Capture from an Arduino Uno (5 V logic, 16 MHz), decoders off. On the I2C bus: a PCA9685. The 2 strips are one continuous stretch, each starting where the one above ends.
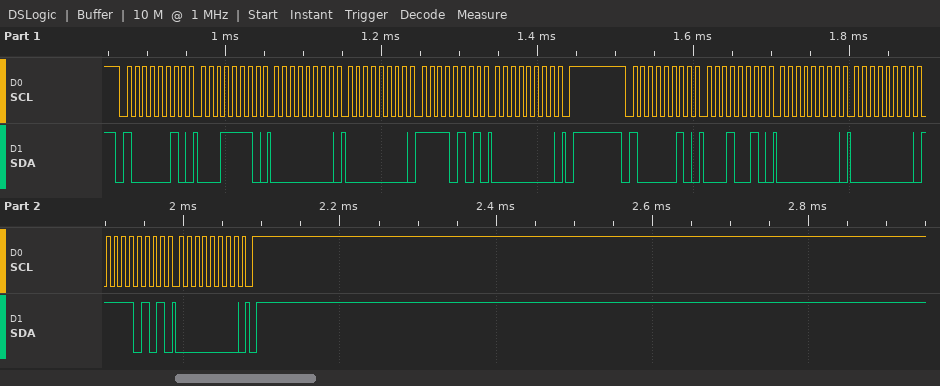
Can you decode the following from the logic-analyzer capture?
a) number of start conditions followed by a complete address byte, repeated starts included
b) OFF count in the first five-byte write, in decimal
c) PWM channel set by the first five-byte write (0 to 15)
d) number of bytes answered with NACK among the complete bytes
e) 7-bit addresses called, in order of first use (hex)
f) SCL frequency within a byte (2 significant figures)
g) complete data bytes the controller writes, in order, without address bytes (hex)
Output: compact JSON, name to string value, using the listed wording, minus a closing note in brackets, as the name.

{"number of start conditions followed by a complete address byte, repeated starts included": "2", "OFF count in the first five-byte write, in decimal": "245", "PWM channel set by the first five-byte write": "6", "number of bytes answered with NACK among the complete bytes": "0", "7-bit addresses called, in order of first use": "0x41", "SCL frequency within a byte": "100 kHz", "complete data bytes the controller writes, in order, without address bytes": "1E 00 00 F5 00 12 00 00 F5 00"}
